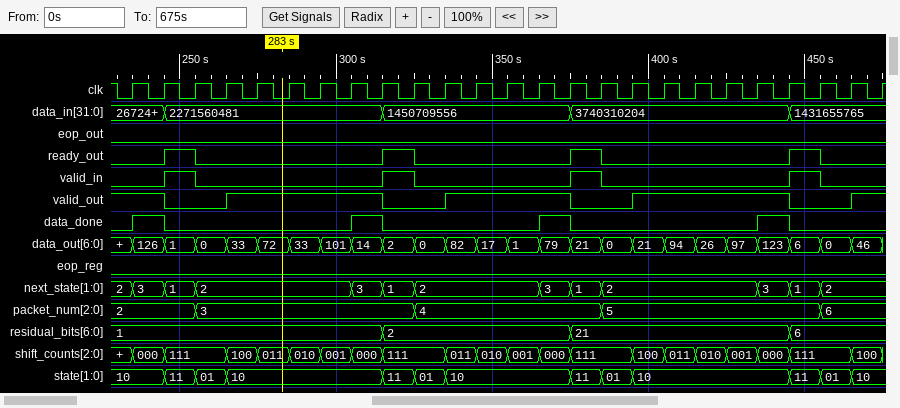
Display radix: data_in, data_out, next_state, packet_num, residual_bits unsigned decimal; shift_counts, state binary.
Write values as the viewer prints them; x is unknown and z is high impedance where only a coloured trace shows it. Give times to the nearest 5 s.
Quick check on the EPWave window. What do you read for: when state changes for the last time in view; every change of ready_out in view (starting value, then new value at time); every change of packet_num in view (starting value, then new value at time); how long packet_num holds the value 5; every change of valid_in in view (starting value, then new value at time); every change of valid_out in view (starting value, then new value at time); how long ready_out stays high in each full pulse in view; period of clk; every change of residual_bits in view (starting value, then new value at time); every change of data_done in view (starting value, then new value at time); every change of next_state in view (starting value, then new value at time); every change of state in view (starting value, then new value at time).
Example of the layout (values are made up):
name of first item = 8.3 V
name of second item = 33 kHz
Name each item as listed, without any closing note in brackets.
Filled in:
when state changes for the last time in view = 465 s
every change of ready_out in view = 0, 1 at 245 s, 0 at 255 s, 1 at 315 s, 0 at 325 s, 1 at 375 s, 0 at 385 s, 1 at 445 s, 0 at 455 s
every change of packet_num in view = 2, 3 at 255 s, 4 at 325 s, 5 at 385 s, 6 at 455 s
how long packet_num holds the value 5 = 70 s
every change of valid_in in view = 0, 1 at 245 s, 0 at 255 s, 1 at 315 s, 0 at 325 s, 1 at 375 s, 0 at 385 s, 1 at 445 s, 0 at 455 s
every change of valid_out in view = 1, 0 at 245 s, 1 at 265 s, 0 at 315 s, 1 at 335 s, 0 at 375 s, 1 at 395 s, 0 at 445 s, 1 at 465 s
how long ready_out stays high in each full pulse in view = 10 s, 10 s, 10 s, 10 s
period of clk = 10 s
every change of residual_bits in view = 1, 2 at 315 s, 21 at 375 s, 6 at 445 s
every change of data_done in view = 0, 1 at 235 s, 0 at 245 s, 1 at 305 s, 0 at 315 s, 1 at 365 s, 0 at 375 s, 1 at 435 s, 0 at 445 s
every change of next_state in view = 2, 3 at 235 s, 1 at 245 s, 2 at 255 s, 3 at 305 s, 1 at 315 s, 2 at 325 s, 3 at 365 s, 1 at 375 s, 2 at 385 s, 3 at 435 s, 1 at 445 s, 2 at 455 s
every change of state in view = 10, 11 at 245 s, 01 at 255 s, 10 at 265 s, 11 at 315 s, 01 at 325 s, 10 at 335 s, 11 at 375 s, 01 at 385 s, 10 at 395 s, 11 at 445 s, 01 at 455 s, 10 at 465 s
